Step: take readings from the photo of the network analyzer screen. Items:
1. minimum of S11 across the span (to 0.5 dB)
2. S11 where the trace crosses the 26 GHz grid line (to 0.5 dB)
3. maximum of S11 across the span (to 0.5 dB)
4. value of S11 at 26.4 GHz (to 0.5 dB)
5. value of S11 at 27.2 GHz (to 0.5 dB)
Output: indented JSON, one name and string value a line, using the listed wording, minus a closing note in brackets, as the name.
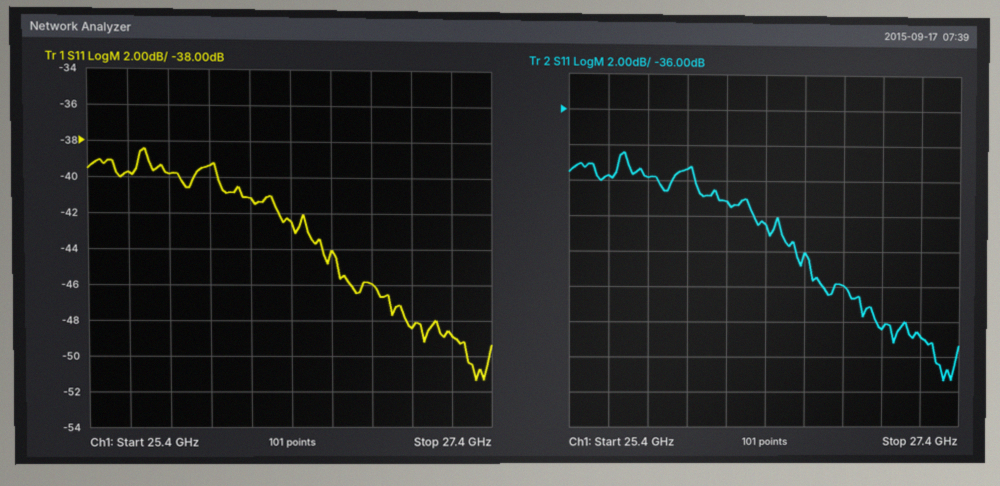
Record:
{
  "minimum of S11 across the span": "-51.5 dB",
  "S11 where the trace crosses the 26 GHz grid line": "-39.5 dB",
  "maximum of S11 across the span": "-38.5 dB",
  "value of S11 at 26.4 GHz": "-42.5 dB",
  "value of S11 at 27.2 GHz": "-49.0 dB"
}
